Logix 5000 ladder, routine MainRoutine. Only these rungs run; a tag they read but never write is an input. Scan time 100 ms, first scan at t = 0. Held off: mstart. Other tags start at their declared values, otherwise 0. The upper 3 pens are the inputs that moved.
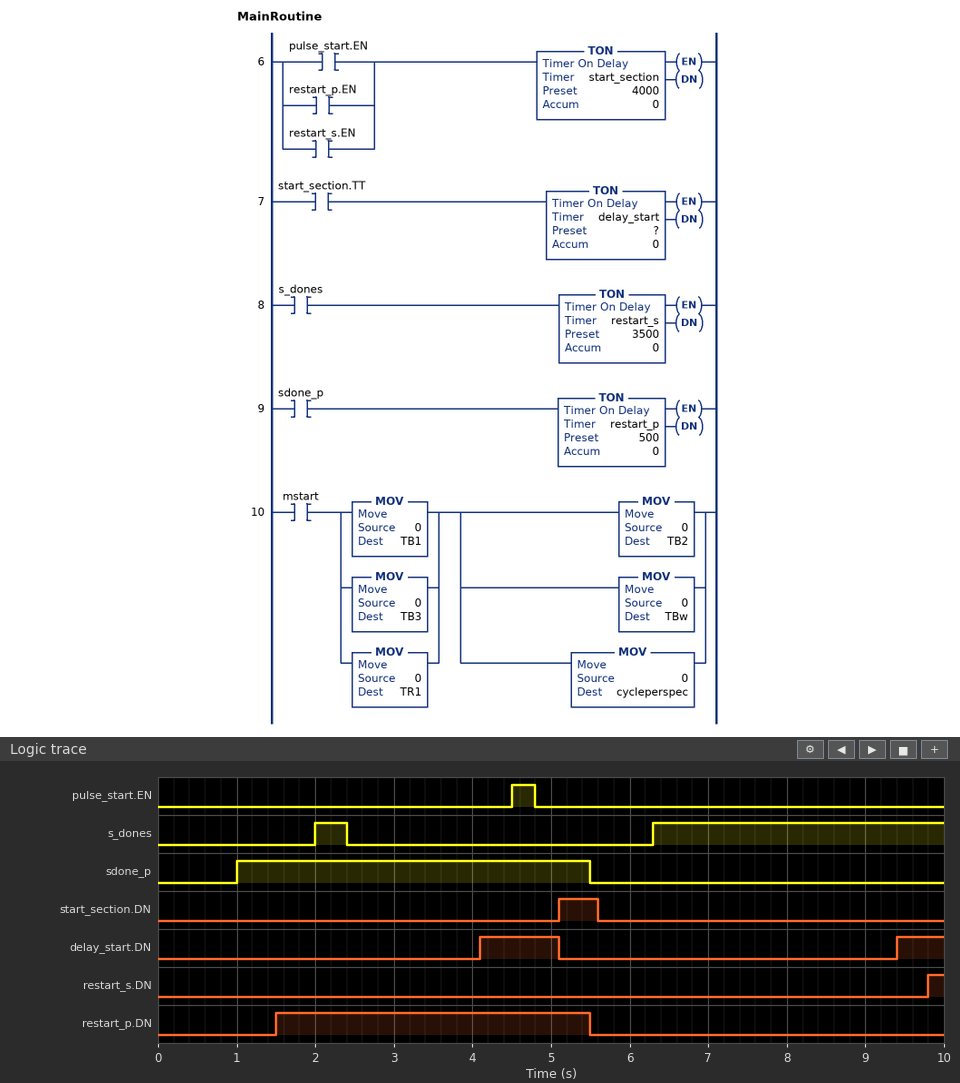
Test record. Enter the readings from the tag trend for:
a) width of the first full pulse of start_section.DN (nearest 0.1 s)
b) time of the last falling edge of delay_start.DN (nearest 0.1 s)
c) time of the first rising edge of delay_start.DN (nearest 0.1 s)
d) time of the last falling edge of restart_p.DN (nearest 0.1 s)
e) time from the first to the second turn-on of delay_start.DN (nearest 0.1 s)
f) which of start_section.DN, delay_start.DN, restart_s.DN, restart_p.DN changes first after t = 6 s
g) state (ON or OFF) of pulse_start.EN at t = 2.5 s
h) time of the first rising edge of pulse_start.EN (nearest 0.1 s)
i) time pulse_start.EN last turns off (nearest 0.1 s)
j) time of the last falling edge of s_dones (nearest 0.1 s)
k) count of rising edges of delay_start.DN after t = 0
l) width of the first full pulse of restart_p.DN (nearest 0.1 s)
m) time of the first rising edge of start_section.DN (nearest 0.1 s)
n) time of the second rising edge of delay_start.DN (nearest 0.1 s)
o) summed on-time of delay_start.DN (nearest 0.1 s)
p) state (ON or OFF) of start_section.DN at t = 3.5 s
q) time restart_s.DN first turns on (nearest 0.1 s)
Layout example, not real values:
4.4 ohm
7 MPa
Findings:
0.5 s
5.1 s
4.1 s
5.5 s
5.3 s
delay_start.DN
OFF
4.5 s
4.8 s
2.4 s
2
4.0 s
5.1 s
9.4 s
1.6 s
OFF
9.8 s
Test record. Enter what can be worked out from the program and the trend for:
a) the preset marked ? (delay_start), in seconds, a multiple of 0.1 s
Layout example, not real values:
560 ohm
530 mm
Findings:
3.0 s
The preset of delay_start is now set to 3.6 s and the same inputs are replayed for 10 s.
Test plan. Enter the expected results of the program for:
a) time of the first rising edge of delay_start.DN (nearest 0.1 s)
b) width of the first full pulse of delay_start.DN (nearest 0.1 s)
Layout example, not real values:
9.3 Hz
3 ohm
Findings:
4.7 s
0.4 s
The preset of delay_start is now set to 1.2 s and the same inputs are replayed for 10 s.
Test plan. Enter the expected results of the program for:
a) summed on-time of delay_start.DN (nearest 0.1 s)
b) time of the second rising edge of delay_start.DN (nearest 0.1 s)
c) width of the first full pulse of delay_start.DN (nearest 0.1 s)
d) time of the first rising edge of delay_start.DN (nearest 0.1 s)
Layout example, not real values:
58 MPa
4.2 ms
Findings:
5.2 s
7.6 s
2.8 s
2.3 s
